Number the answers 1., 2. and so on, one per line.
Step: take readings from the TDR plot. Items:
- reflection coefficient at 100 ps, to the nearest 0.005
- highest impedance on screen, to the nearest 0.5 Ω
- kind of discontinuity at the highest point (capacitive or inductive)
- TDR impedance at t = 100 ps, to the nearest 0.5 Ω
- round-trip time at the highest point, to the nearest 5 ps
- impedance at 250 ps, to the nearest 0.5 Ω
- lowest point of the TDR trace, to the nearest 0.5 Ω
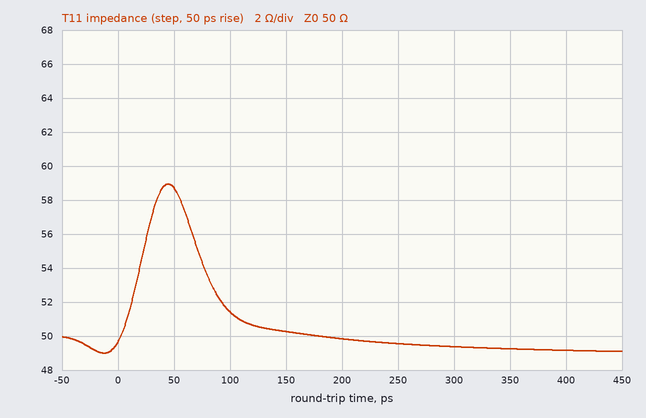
1. +0.015
2. 59.0 Ω
3. inductive
4. 51.5 Ω
5. 45 ps
6. 49.5 Ω
7. 49.0 Ω
